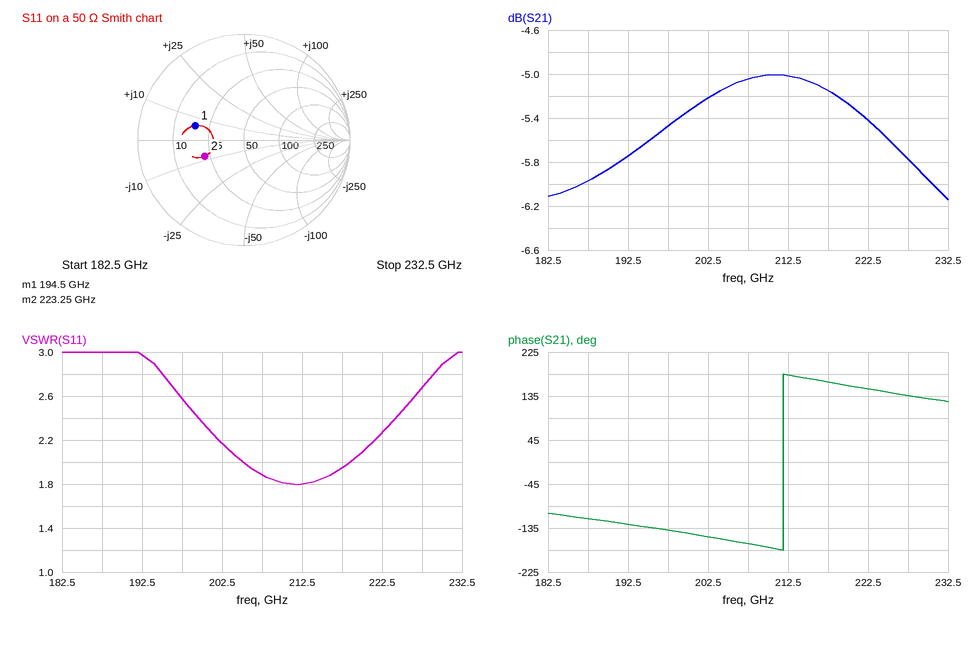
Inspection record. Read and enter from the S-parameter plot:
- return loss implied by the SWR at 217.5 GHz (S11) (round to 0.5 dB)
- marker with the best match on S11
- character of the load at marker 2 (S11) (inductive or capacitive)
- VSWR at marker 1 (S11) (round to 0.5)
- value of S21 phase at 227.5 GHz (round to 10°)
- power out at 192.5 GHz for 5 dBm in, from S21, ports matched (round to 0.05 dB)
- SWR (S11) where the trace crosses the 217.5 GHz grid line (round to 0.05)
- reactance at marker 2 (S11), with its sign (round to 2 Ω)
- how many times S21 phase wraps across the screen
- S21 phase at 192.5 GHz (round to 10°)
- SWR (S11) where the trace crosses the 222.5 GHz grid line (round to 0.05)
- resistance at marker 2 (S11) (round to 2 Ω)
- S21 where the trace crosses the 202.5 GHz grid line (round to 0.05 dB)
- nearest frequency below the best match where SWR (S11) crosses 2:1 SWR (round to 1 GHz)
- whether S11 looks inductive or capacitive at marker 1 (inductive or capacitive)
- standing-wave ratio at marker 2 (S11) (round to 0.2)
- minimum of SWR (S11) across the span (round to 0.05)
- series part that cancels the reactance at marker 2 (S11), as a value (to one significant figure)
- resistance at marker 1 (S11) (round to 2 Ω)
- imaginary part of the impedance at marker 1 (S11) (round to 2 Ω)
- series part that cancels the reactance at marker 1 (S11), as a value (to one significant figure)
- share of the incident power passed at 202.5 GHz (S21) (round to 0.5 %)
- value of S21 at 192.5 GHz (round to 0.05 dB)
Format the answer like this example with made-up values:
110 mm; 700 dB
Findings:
10.0 dB; marker 2; capacitive; 3.0; 140°; -0.75 dBm; 1.95; -8 Ω; 1; -130°; 2.25; 22 Ω; -5.20 dB; 205 GHz; inductive; 2.4; 1.80; 6 pH; 18 Ω; +6 Ω; 100 fF; 30.0 %; -5.75 dB
